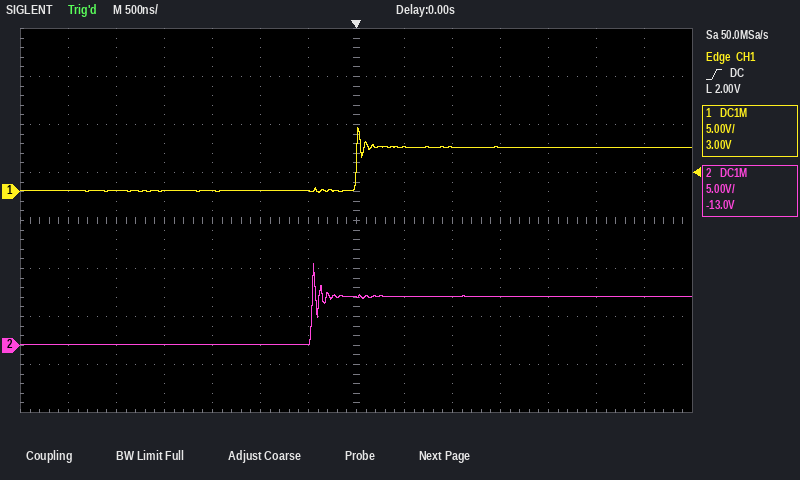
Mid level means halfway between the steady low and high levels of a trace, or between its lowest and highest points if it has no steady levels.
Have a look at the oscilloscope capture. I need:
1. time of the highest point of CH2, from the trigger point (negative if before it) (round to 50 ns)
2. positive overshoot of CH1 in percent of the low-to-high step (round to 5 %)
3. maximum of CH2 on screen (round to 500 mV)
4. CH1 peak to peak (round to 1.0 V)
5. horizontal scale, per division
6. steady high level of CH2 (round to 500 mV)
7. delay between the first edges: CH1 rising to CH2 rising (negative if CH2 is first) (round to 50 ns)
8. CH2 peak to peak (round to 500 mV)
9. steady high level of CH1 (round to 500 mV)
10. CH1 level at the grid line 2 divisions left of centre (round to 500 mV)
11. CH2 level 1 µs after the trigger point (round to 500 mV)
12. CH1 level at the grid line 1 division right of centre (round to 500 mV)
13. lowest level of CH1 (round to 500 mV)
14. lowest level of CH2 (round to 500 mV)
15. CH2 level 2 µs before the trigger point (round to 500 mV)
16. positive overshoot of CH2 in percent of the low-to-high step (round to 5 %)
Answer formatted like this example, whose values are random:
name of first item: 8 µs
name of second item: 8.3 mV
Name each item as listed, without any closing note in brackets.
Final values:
time of the highest point of CH2, from the trigger point (negative if before it): -450 ns
positive overshoot of CH1 in percent of the low-to-high step: 45 %
maximum of CH2 on screen: 8.5 V
CH1 peak to peak: 7.0 V
horizontal scale, per division: 500 ns
steady high level of CH2: 5.0 V
delay between the first edges: CH1 rising to CH2 rising (negative if CH2 is first): -450 ns
CH2 peak to peak: 8.5 V
steady high level of CH1: 4.5 V
CH1 level at the grid line 2 divisions left of centre: 0.0 V
CH2 level 1 µs after the trigger point: 5.0 V
CH1 level at the grid line 1 division right of centre: 4.5 V
lowest level of CH1: 0.0 V
lowest level of CH2: 0.0 V
CH2 level 2 µs before the trigger point: 0.0 V
positive overshoot of CH2 in percent of the low-to-high step: 70 %
